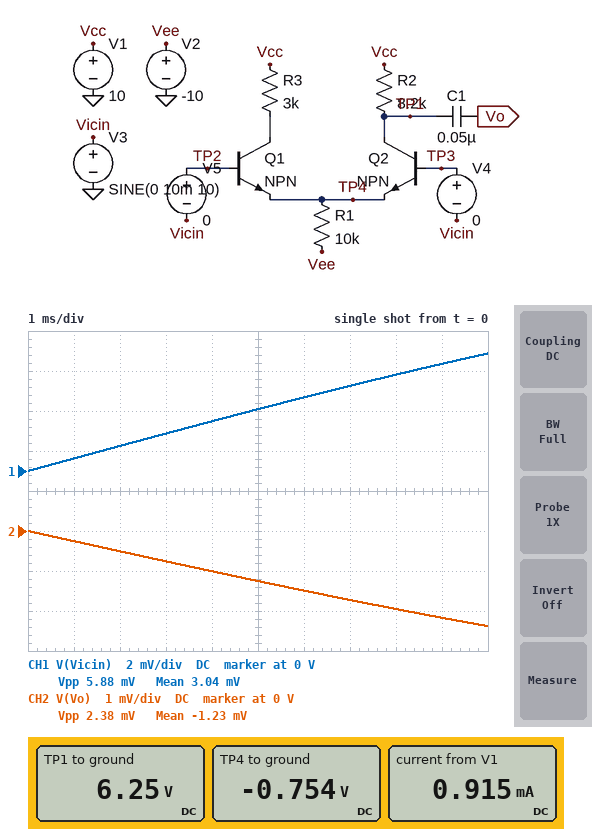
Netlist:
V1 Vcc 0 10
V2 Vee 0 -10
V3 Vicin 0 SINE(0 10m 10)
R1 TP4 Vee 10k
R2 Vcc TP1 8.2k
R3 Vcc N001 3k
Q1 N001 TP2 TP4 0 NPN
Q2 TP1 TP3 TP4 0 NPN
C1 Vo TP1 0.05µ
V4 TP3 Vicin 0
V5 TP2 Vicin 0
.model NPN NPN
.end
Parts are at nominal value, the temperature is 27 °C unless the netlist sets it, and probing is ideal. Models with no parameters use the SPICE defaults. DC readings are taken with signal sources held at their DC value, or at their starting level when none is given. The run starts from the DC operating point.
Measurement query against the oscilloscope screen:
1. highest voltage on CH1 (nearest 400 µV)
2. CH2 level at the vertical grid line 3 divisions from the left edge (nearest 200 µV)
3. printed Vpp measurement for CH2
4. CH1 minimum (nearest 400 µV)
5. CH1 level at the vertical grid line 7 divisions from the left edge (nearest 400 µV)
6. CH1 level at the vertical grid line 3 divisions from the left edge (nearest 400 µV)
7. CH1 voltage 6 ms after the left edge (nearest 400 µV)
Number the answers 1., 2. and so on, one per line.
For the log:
1. 6.0 mV
2. -800 µV
3. 2.38 mV
4. 0 V
5. 4.4 mV
6. 2.0 mV
7. 3.6 mV
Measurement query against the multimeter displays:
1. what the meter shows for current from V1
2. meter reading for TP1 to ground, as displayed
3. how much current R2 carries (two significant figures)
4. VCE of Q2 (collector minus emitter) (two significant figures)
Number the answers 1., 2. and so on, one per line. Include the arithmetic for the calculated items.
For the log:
1. 0.915 mA
2. 6.25 V
3. (10 V - 6.25 V) / 8.2 kΩ = 460 µA
4. 6.25 V - (-754 mV) = 7.0 V
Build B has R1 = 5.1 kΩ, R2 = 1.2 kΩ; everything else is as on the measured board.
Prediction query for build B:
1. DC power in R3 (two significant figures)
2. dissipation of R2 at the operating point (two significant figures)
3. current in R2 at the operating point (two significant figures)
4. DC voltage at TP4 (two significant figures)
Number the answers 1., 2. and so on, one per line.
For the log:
1. 2.4 mW
2. 960 µW
3. 900 µA
4. -770 mV
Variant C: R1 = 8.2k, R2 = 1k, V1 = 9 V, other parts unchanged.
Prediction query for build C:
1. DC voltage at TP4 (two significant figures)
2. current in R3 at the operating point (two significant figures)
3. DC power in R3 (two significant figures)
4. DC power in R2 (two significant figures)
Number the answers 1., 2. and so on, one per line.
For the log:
1. -760 mV
2. 560 µA
3. 930 µW
4. 310 µW
